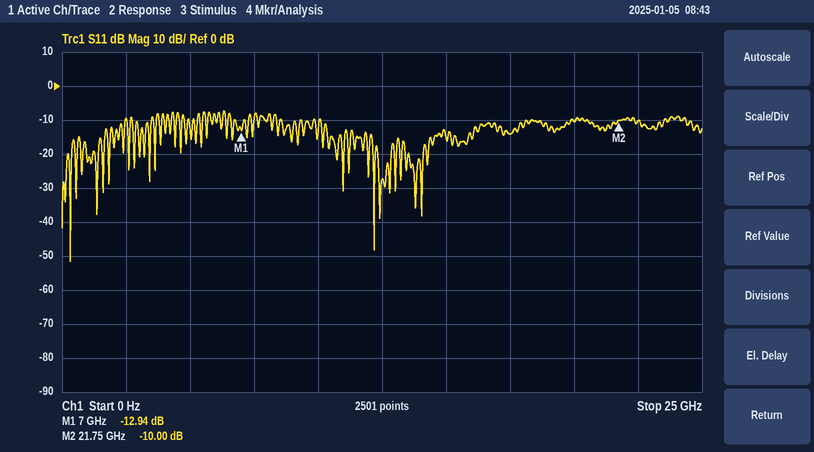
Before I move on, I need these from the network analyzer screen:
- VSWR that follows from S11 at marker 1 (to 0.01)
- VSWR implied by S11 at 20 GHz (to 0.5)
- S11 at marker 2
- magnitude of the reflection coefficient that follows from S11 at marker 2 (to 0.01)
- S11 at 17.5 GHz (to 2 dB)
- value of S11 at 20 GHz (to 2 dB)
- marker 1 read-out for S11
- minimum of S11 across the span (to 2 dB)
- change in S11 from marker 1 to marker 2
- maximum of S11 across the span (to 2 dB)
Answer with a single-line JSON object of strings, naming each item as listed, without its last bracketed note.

{"VSWR that follows from S11 at marker 1": "1.58", "VSWR implied by S11 at 20 GHz": "2.0", "S11 at marker 2": "-10.00 dB", "magnitude of the reflection coefficient that follows from S11 at marker 2": "0.32", "S11 at 17.5 GHz": "-14 dB", "value of S11 at 20 GHz": "-10 dB", "marker 1 read-out for S11": "-12.94 dB", "minimum of S11 across the span": "-52 dB", "change in S11 from marker 1 to marker 2": "2.94 dB", "maximum of S11 across the span": "-8 dB"}
